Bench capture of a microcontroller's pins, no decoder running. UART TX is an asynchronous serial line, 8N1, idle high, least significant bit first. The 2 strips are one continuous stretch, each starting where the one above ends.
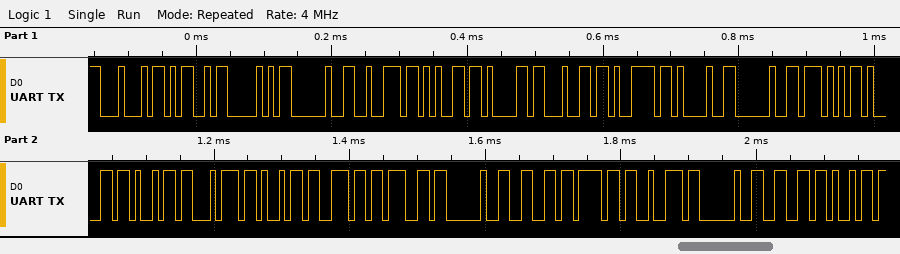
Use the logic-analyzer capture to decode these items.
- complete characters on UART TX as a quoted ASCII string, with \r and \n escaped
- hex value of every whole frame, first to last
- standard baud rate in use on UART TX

"DMP ready! Waiting for fi"
44 4D 50 20 72 65 61 64 79 21 20 57 61 69 74 69 6E 67 20 66 6F 72 20 66 69
115200 baud
